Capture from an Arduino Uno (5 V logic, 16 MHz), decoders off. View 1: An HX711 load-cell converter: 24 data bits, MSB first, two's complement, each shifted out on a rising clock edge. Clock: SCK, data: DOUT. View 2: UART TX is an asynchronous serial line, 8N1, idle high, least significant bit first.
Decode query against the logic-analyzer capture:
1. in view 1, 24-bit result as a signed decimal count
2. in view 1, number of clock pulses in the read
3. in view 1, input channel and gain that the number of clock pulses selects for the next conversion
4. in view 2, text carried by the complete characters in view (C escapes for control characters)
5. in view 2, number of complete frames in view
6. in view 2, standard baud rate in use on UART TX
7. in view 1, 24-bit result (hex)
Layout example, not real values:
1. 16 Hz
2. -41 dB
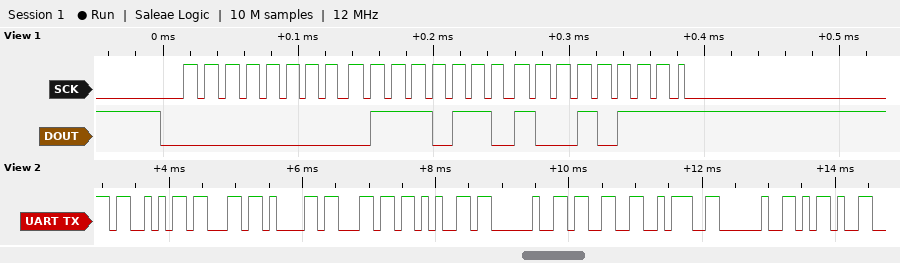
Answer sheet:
1. 30359
2. 25
3. channel A, gain 128
4. "Scale 3: -"
5. 10
6. 9600 baud
7. 0x007697
